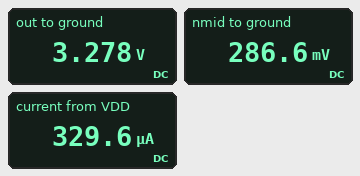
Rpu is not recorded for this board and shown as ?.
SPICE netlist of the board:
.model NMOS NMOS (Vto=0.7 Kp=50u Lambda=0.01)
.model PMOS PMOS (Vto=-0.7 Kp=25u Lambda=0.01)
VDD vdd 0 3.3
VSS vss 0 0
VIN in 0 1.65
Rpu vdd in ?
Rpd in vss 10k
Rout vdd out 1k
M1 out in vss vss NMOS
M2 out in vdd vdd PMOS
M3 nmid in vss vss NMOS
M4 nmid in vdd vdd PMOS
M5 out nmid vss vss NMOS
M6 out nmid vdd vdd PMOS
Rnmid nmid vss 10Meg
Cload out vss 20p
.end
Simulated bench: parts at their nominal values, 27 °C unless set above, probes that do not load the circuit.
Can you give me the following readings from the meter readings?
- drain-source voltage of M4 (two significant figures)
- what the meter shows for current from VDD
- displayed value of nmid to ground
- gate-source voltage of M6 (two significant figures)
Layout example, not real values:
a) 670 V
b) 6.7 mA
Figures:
a) -3.0 V
b) 329.6 µA
c) 286.6 mV
d) -3.0 V
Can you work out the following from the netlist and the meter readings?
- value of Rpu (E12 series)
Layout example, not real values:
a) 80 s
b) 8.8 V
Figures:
a) 5.6 kΩ
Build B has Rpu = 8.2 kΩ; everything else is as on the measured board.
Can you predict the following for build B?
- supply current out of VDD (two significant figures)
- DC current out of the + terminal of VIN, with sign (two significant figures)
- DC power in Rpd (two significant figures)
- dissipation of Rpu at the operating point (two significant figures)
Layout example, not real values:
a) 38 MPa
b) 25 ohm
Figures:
a) 240 µA
b) -36 µA
c) 270 µW
d) 330 µW
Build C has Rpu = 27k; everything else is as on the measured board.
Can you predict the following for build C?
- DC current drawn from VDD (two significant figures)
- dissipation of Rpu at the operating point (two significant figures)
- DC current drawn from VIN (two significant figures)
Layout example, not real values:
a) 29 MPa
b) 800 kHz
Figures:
a) 96 µA
b) 100 µW
c) 100 µA
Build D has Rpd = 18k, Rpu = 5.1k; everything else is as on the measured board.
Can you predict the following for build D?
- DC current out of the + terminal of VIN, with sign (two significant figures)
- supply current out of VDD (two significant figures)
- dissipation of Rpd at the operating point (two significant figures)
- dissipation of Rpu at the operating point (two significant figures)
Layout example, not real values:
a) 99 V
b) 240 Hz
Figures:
a) -230 µA
b) 360 µA
c) 150 µW
d) 530 µW
